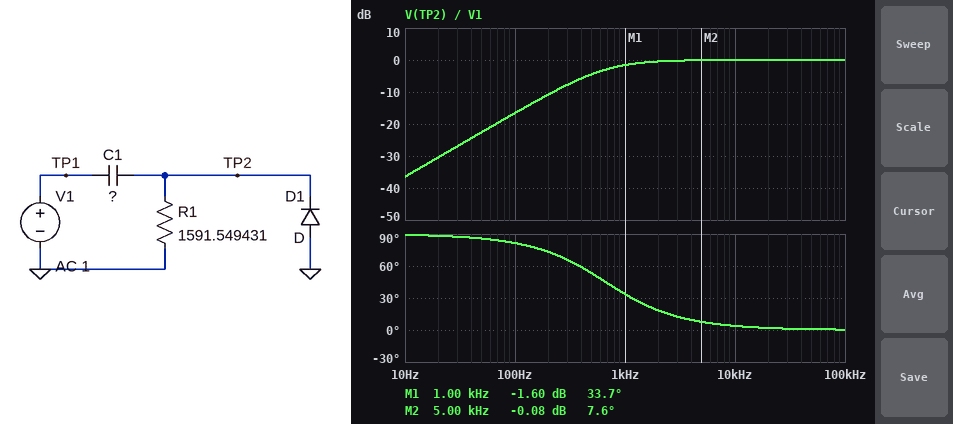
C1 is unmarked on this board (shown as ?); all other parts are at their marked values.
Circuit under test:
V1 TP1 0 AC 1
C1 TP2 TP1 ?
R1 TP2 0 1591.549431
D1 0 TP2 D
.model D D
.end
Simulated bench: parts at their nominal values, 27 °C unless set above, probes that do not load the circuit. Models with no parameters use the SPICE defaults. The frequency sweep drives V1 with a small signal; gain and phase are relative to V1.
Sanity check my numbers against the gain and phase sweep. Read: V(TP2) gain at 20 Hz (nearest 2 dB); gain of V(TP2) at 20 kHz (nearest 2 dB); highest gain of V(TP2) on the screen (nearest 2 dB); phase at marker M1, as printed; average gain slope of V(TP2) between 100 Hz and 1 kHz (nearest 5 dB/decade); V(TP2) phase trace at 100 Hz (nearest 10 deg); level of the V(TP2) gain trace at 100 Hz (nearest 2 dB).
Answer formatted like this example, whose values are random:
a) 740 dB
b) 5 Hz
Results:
a) -30 dB
b) 0 dB
c) 0 dB
d) 33.7 deg
e) 15 dB/decade
f) 80 deg
g) -16 dB
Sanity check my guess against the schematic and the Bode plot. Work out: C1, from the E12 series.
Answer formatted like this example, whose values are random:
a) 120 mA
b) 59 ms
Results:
a) 150 nF
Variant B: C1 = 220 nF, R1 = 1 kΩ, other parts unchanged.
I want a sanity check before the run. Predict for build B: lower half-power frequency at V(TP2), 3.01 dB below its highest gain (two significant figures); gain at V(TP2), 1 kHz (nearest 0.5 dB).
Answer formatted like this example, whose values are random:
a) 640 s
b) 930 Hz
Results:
a) 720 Hz
b) -2.0 dB
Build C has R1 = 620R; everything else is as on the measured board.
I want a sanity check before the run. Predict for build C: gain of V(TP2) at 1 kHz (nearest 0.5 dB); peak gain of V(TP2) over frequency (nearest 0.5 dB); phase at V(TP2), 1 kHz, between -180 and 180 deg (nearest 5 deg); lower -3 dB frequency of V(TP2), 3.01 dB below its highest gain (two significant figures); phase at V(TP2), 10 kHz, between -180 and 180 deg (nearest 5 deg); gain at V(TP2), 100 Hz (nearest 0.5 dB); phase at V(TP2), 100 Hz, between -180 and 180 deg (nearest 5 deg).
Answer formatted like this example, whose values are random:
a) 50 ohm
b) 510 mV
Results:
a) -6.0 dB
b) 0 dB
c) 60 deg
d) 1.7 kHz
e) 10 deg
f) -24.5 dB
g) 85 deg
